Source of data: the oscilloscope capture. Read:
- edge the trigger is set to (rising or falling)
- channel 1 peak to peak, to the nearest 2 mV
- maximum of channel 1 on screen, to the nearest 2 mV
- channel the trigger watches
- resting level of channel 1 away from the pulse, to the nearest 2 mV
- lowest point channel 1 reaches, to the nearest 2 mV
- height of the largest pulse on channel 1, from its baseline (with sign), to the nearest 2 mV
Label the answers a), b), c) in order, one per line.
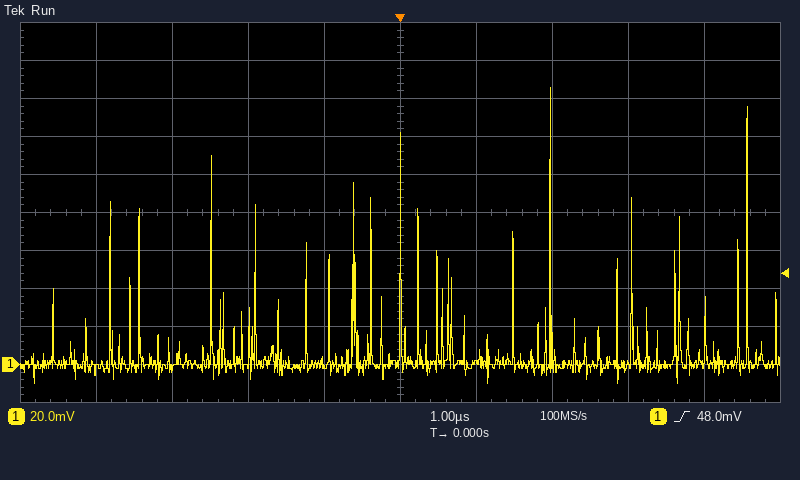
a) rising
b) 156 mV
c) 146 mV
d) channel 1
e) 0 mV
f) -10 mV
g) +146 mV
